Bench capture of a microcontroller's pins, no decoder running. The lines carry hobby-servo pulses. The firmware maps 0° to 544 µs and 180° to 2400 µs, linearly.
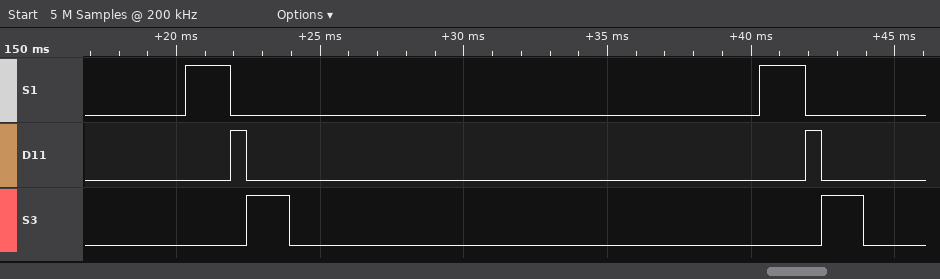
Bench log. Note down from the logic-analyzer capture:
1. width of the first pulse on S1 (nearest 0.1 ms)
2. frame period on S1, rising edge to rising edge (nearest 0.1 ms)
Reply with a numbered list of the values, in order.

1. 1.6 ms
2. 20.0 ms
